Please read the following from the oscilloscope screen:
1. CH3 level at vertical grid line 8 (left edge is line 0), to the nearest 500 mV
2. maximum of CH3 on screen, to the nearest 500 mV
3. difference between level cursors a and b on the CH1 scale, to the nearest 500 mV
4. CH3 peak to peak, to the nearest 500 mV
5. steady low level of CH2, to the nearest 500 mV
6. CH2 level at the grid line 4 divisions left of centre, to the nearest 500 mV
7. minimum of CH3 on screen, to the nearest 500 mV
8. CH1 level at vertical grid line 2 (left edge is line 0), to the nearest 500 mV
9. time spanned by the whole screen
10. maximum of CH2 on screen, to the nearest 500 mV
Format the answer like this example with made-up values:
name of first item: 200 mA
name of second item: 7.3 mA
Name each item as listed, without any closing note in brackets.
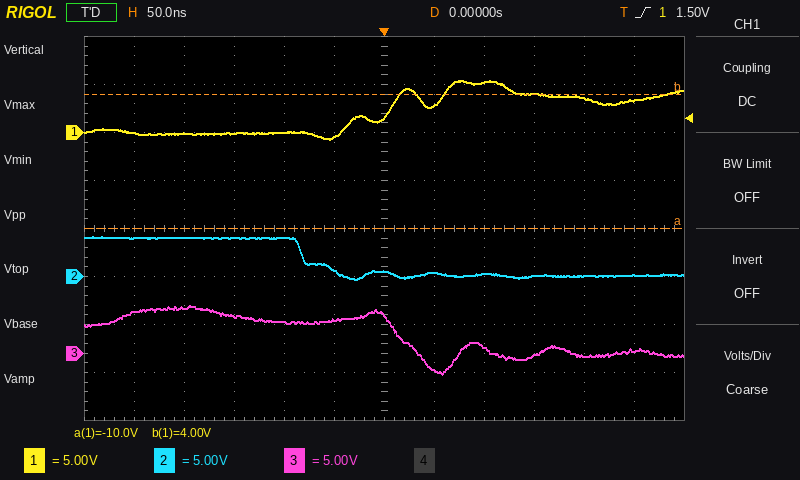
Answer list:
CH3 level at vertical grid line 8 (left edge is line 0), to the nearest 500 mV: 500 mV
maximum of CH3 on screen, to the nearest 500 mV: 5.0 V
difference between level cursors a and b on the CH1 scale, to the nearest 500 mV: 14.0 V
CH3 peak to peak, to the nearest 500 mV: 7.0 V
steady low level of CH2, to the nearest 500 mV: 0.0 V
CH2 level at the grid line 4 divisions left of centre, to the nearest 500 mV: 4.0 V
minimum of CH3 on screen, to the nearest 500 mV: -2.0 V
CH1 level at vertical grid line 2 (left edge is line 0), to the nearest 500 mV: 0.0 V
time spanned by the whole screen: 600 ns
maximum of CH2 on screen, to the nearest 500 mV: 4.0 V
